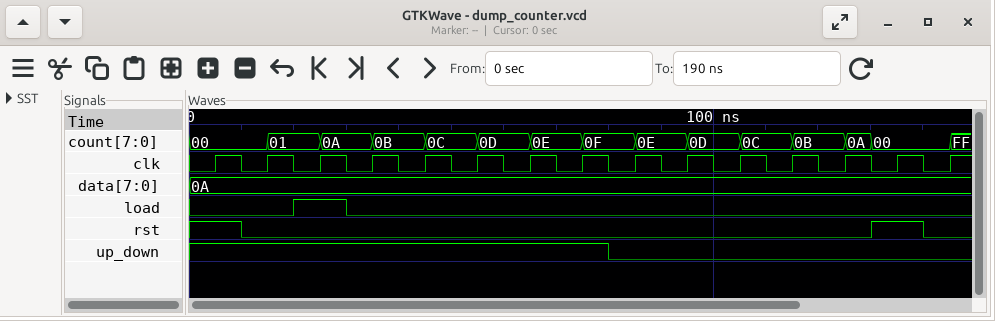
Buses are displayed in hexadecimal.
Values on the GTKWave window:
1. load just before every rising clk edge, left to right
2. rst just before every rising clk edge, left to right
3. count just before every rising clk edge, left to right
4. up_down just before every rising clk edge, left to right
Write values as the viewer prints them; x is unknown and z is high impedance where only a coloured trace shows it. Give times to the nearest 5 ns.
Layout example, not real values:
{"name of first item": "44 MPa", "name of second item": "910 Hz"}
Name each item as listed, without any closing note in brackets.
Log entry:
{"load just before every rising clk edge, left to right": "0 0 1 0 0 0 0 0 0 0 0 0 0 0 0", "rst just before every rising clk edge, left to right": "1 0 0 0 0 0 0 0 0 0 0 0 0 1 0", "count just before every rising clk edge, left to right": "00, 00, 01, 0A, 0B, 0C, 0D, 0E, 0F, 0E, 0D, 0C, 0B, 00, 00", "up_down just before every rising clk edge, left to right": "1 1 1 1 1 1 1 1 0 0 0 0 0 0 0"}
